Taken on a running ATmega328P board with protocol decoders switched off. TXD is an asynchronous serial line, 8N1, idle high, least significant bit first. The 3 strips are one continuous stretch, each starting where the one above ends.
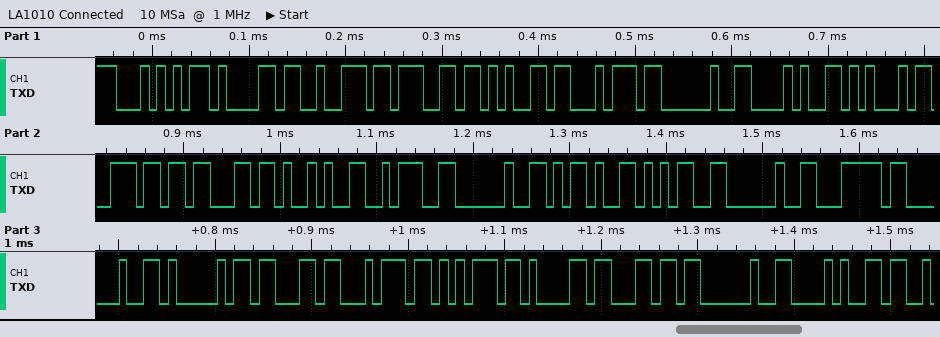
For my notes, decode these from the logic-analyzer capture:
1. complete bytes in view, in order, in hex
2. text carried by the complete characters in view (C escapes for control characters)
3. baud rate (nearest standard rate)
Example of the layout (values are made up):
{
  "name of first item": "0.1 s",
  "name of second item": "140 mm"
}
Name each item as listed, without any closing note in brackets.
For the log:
{
  "complete bytes in view, in order, in hex": "54 61 72 67 65 74 20 28 45 6E 63 29 3A 20 2D 35 20 7C 20 41 63 74 75 61 6C 20 28",
  "text carried by the complete characters in view": "\"Target (Enc): -5 | Actual (\"",
  "baud rate": "115200 baud"
}
